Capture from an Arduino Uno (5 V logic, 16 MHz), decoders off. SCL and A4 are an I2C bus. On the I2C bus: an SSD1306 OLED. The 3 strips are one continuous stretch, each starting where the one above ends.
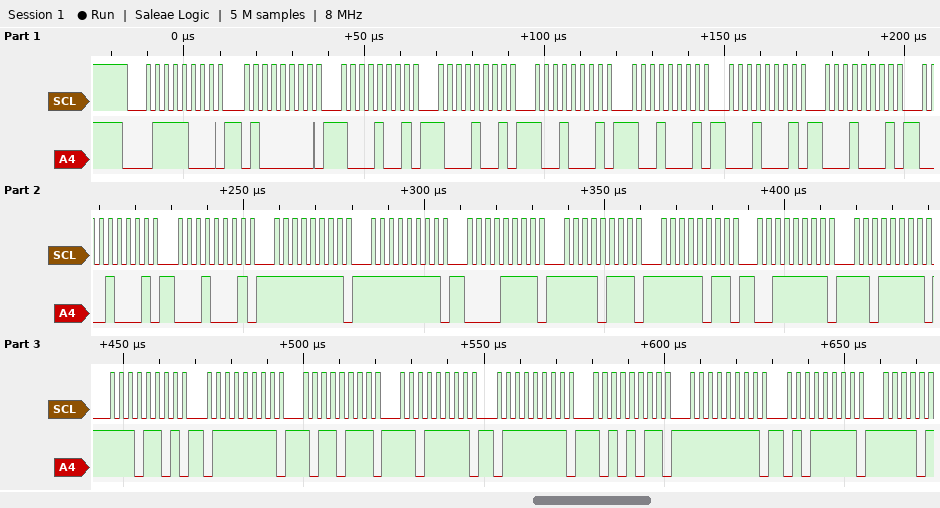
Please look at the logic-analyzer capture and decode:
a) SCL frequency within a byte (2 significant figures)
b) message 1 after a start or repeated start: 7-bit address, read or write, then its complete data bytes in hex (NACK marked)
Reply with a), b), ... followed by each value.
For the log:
a) 400 kHz
b) 0x3C write: 40 89 89 91 91 11 11 11 11 FF FF 0F F7 FB 3F DF ED 7F B7 DF 7F AB FF 5F
